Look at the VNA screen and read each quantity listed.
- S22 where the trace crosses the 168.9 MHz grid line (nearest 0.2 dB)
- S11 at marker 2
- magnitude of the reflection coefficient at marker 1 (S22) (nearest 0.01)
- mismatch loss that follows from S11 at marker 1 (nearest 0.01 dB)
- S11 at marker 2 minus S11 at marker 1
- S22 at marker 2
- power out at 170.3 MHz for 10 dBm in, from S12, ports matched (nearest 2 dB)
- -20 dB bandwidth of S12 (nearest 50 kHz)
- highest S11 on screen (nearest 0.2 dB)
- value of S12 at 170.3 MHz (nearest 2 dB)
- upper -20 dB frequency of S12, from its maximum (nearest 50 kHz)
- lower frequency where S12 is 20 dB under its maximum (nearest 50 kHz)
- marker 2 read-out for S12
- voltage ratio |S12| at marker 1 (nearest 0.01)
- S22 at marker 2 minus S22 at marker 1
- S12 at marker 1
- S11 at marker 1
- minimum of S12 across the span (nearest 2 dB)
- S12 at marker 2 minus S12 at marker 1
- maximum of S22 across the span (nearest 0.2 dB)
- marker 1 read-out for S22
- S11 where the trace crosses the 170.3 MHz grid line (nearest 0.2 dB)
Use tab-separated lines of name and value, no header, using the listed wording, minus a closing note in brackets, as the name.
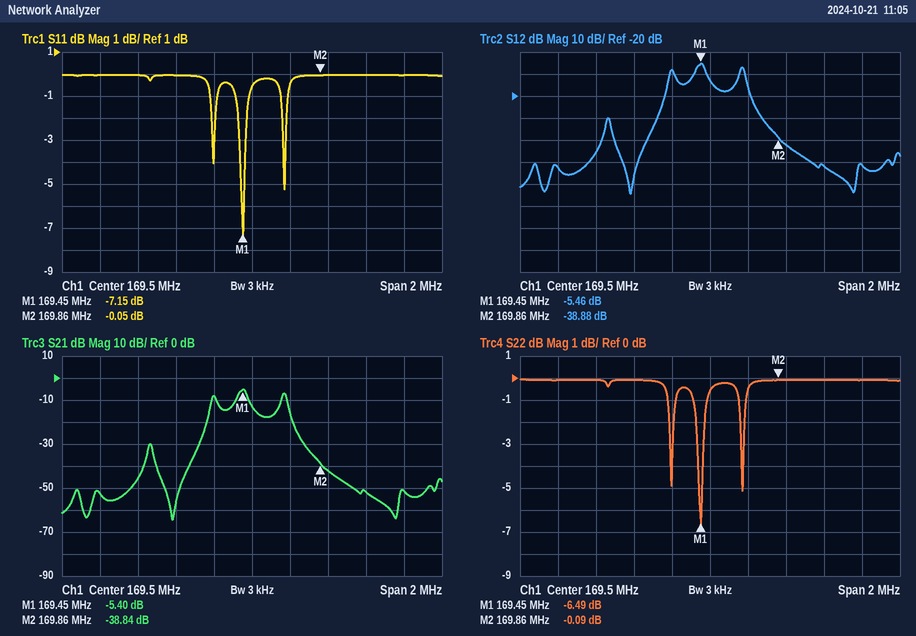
S22 where the trace crosses the 168.9 MHz grid line	0.0 dB
S11 at marker 2	-0.05 dB
magnitude of the reflection coefficient at marker 1 (S22)	0.47
mismatch loss that follows from S11 at marker 1	0.93 dB
S11 at marker 2 minus S11 at marker 1	7.10 dB
S22 at marker 2	-0.09 dB
power out at 170.3 MHz for 10 dBm in, from S12, ports matched	-42 dBm
-20 dB bandwidth of S12	500 kHz
highest S11 on screen	0.0 dB
value of S12 at 170.3 MHz	-52 dB
upper -20 dB frequency of S12, from its maximum	169.75 MHz
lower frequency where S12 is 20 dB under its maximum	169.25 MHz
marker 2 read-out for S12	-38.88 dB
voltage ratio |S12| at marker 1	0.53
S22 at marker 2 minus S22 at marker 1	6.40 dB
S12 at marker 1	-5.46 dB
S11 at marker 1	-7.15 dB
minimum of S12 across the span	-64 dB
S12 at marker 2 minus S12 at marker 1	-33.42 dB
maximum of S22 across the span	0.0 dB
marker 1 read-out for S22	-6.49 dB
S11 where the trace crosses the 170.3 MHz grid line	0.0 dB
